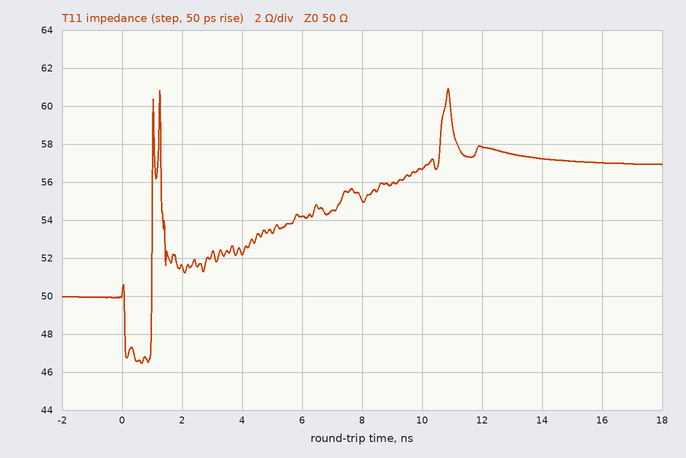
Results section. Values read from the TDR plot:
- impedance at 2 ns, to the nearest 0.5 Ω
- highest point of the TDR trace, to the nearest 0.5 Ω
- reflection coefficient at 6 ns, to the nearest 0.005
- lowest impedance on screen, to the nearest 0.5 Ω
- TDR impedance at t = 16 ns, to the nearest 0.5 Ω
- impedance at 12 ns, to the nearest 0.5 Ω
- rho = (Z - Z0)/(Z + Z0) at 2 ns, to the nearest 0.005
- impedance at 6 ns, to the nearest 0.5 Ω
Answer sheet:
51.5 Ω
61.0 Ω
+0.040
46.5 Ω
57.0 Ω
58.0 Ω
+0.015
54.0 Ω
